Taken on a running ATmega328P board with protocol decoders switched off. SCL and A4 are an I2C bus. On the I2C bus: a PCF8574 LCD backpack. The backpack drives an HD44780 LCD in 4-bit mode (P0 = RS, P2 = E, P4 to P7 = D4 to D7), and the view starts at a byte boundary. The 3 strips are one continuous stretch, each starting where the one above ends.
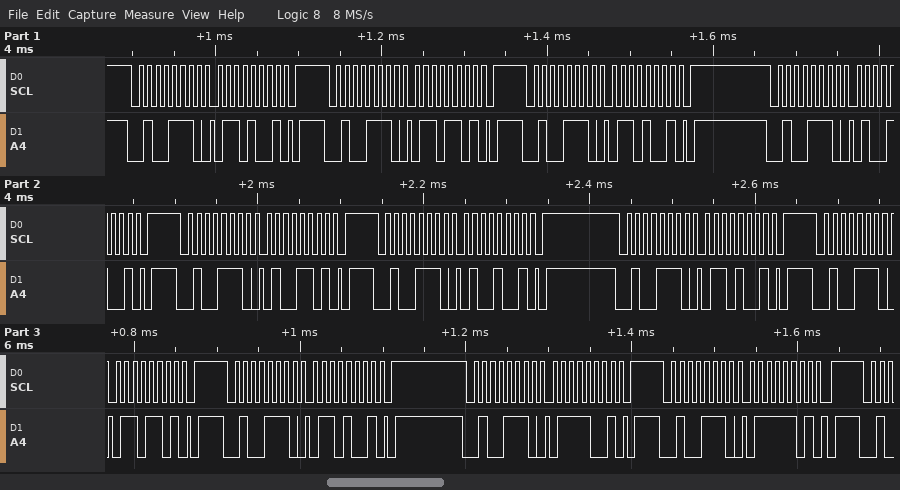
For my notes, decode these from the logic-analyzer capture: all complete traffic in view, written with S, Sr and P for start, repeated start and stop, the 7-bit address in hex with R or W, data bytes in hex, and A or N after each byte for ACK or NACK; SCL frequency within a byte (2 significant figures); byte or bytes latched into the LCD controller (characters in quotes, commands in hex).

S 27W A 69 A P S 27W A 6D A P S 27W A 69 A P S 27W A 49 A P S 27W A 4D A P S 27W A 49 A P S 27W A 69 A P S 27W A 6D A P S 27W A 69 A P S 27W A 79 A P S 27W A 7D A P
100 kHz
'd'
